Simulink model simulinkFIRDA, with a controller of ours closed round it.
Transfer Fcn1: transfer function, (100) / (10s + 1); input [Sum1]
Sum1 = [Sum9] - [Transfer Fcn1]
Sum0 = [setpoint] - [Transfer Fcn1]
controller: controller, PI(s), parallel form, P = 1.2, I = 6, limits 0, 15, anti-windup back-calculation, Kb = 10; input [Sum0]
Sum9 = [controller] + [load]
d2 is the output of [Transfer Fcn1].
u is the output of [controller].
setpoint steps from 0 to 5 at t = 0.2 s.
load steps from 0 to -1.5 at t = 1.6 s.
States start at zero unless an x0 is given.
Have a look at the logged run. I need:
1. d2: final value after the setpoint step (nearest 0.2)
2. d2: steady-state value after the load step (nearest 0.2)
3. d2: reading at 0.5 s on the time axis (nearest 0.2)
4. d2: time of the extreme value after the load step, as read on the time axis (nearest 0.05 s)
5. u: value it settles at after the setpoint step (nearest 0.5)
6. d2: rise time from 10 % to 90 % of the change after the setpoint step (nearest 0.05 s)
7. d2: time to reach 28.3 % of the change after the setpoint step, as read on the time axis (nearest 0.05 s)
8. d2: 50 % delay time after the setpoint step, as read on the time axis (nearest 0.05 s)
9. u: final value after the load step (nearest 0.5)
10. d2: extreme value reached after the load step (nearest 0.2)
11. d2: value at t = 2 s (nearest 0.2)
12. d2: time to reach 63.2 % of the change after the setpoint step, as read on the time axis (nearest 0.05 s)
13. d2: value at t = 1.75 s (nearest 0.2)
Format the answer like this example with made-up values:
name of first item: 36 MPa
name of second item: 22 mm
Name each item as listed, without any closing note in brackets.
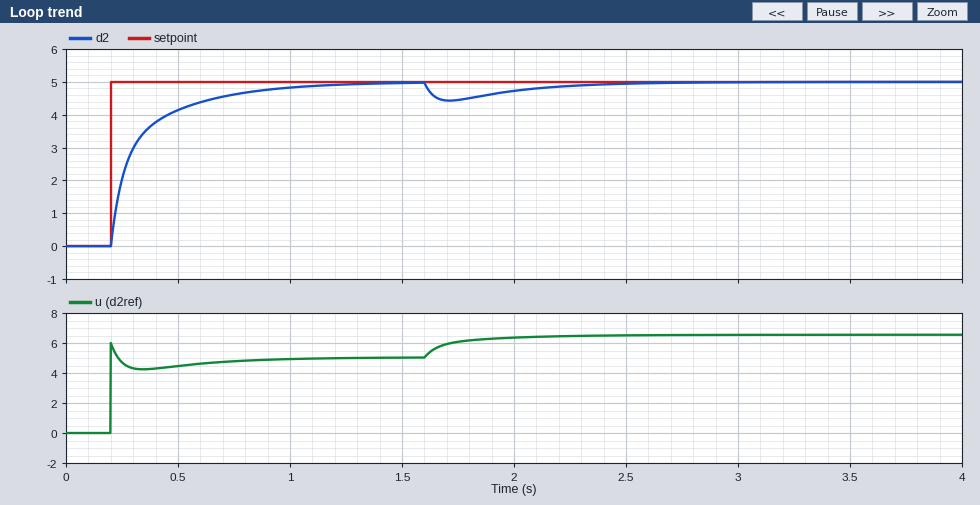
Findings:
d2: final value after the setpoint step: 5.0
d2: steady-state value after the load step: 5.0
d2: reading at 0.5 s on the time axis: 4.2
d2: time of the extreme value after the load step, as read on the time axis: 1.70 s
u: value it settles at after the setpoint step: 5.0
d2: rise time from 10 % to 90 % of the change after the setpoint step: 0.45 s
d2: time to reach 28.3 % of the change after the setpoint step, as read on the time axis: 0.25 s
d2: 50 % delay time after the setpoint step, as read on the time axis: 0.25 s
u: final value after the load step: 6.5
d2: extreme value reached after the load step: 4.4
d2: value at t = 2 s: 4.8
d2: time to reach 63.2 % of the change after the setpoint step, as read on the time axis: 0.30 s
d2: value at t = 1.75 s: 4.4
